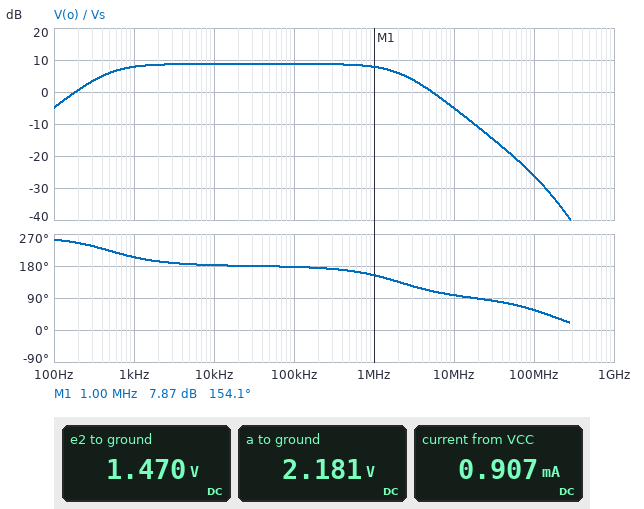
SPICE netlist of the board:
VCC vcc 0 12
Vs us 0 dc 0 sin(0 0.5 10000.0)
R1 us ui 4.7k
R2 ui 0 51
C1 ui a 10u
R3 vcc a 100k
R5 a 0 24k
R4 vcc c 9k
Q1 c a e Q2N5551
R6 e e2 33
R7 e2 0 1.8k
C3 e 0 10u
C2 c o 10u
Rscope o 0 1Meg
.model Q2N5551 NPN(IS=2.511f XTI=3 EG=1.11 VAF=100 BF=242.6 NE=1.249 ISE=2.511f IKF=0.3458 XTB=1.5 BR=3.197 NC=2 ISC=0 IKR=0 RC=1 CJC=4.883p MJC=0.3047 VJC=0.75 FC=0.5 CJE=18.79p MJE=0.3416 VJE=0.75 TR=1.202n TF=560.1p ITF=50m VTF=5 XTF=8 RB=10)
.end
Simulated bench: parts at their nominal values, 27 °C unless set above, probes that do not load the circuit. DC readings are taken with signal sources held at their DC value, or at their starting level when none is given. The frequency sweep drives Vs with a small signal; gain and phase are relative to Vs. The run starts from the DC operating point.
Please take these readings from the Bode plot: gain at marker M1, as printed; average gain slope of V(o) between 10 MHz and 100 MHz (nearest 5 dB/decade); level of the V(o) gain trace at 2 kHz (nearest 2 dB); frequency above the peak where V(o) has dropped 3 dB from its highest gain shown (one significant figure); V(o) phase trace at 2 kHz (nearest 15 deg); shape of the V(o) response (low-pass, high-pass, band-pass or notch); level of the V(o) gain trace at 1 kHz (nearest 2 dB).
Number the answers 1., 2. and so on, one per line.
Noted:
1. 7.87 dB
2. -20 dB/decade
3. 8 dB
4. 2 MHz
5. 195 deg
6. band-pass
7. 8 dB
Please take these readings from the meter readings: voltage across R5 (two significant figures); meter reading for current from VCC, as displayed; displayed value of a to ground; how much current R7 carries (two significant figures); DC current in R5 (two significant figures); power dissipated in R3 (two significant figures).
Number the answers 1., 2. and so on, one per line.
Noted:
1. 2.2 V
2. 0.907 mA
3. 2.181 V
4. 820 µA
5. 91 µA
6. 960 µW
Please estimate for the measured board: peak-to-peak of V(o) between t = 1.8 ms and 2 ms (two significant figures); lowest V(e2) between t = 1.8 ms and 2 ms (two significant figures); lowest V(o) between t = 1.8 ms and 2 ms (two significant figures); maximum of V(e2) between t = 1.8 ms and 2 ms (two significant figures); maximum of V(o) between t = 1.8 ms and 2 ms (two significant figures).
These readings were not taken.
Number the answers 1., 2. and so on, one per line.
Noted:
1. 2.7 V
2. 1.5 V
3. -1.4 V
4. 1.5 V
5. 1.3 V
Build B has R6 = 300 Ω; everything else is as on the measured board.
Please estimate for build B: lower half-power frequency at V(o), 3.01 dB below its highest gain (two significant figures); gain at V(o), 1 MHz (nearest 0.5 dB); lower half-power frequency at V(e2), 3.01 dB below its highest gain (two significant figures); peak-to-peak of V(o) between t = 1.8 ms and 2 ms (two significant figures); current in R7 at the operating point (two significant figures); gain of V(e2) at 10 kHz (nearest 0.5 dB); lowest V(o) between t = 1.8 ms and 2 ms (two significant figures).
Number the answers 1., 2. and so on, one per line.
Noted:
1. 420 Hz
2. 7.0 dB
3. 870 mHz
4. 2.4 V
5. 720 µA
6. -68.5 dB
7. -1.3 V
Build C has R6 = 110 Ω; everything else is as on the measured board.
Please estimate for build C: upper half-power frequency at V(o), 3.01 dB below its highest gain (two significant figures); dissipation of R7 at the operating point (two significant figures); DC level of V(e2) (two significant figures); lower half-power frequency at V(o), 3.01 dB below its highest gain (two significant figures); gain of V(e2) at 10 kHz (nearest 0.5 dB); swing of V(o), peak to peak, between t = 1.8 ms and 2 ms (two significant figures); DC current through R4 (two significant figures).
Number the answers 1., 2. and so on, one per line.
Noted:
1. 2.2 MHz
2. 1.1 mW
3. 1.4 V
4. 460 Hz
5. -67.0 dB
6. 2.6 V
7. 780 µA
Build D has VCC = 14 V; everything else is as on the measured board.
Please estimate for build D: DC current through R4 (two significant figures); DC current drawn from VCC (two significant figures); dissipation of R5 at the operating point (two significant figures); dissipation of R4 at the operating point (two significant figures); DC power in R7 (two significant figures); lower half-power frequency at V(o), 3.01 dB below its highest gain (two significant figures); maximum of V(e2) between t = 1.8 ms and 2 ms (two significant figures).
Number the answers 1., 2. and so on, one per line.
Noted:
1. 1.0 mA
2. 1.1 mA
3. 270 µW
4. 9.0 mW
5. 1.8 mW
6. 570 Hz
7. 1.8 V
